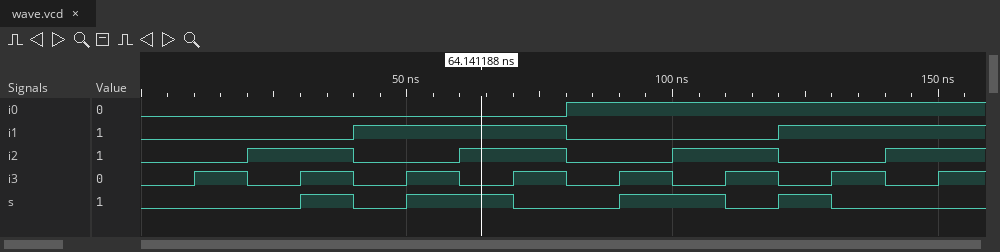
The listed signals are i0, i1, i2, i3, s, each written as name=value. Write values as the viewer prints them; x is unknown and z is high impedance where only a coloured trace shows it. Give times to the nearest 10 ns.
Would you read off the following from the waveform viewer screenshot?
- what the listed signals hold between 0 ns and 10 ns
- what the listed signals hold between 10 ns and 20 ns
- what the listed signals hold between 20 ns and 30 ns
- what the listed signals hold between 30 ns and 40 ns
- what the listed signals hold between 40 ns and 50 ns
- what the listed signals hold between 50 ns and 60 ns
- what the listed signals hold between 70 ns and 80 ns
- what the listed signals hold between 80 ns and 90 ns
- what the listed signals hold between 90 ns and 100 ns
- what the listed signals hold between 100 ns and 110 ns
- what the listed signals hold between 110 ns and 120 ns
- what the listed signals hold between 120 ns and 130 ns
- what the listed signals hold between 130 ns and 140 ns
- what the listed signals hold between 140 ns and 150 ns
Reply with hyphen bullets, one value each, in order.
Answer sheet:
- i0=0, i1=0, i2=0, i3=0, s=0
- i0=0, i1=0, i2=0, i3=1, s=0
- i0=0, i1=0, i2=1, i3=0, s=0
- i0=0, i1=0, i2=1, i3=1, s=1
- i0=0, i1=1, i2=0, i3=0, s=0
- i0=0, i1=1, i2=0, i3=1, s=1
- i0=0, i1=1, i2=1, i3=1, s=0
- i0=1, i1=0, i2=0, i3=0, s=0
- i0=1, i1=0, i2=0, i3=1, s=1
- i0=1, i1=0, i2=1, i3=0, s=1
- i0=1, i1=0, i2=1, i3=1, s=0
- i0=1, i1=1, i2=0, i3=0, s=1
- i0=1, i1=1, i2=0, i3=1, s=0
- i0=1, i1=1, i2=1, i3=0, s=0
